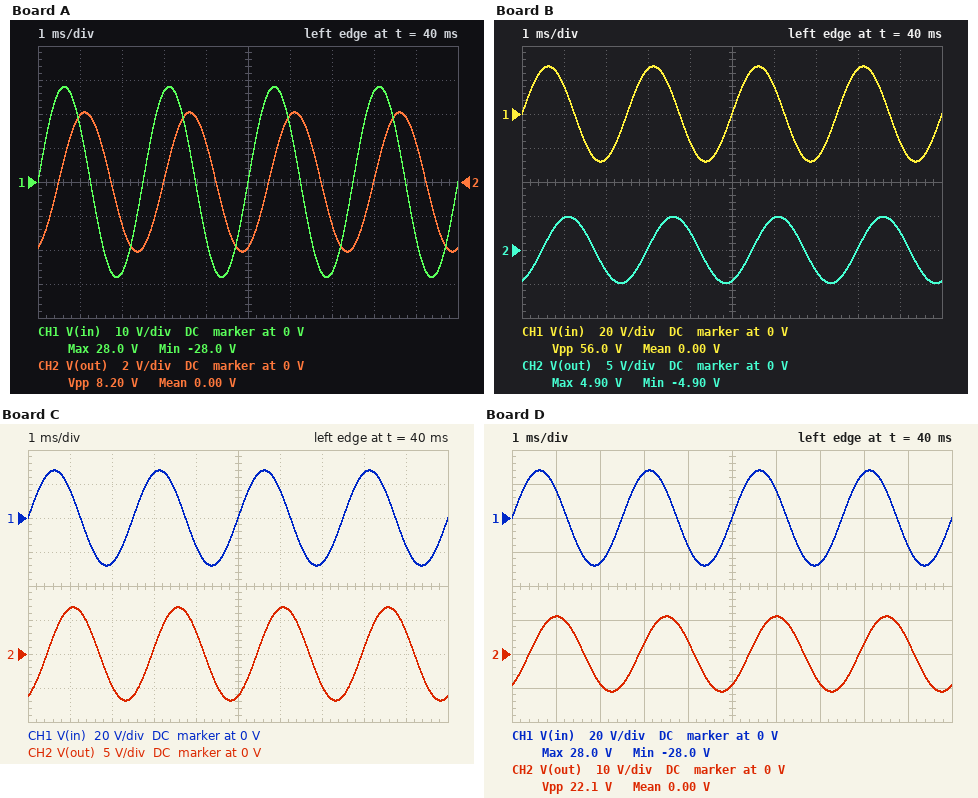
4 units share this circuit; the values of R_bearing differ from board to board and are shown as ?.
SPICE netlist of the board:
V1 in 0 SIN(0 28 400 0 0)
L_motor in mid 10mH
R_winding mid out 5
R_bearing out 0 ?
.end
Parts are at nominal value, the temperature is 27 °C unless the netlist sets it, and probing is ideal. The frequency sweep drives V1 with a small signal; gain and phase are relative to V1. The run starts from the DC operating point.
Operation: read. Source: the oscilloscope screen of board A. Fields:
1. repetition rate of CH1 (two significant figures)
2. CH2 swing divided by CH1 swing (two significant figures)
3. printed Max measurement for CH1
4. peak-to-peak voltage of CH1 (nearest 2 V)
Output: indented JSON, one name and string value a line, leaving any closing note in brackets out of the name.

{
  "repetition rate of CH1": "400 Hz",
  "CH2 swing divided by CH1 swing": "0.15",
  "printed Max measurement for CH1": "28.0 V",
  "peak-to-peak voltage of CH1": "56 V"
}
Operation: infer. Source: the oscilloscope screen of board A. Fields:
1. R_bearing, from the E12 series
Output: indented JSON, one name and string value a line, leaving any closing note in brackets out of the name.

{
  "R_bearing, from the E12 series": "3.9 Ω"
}
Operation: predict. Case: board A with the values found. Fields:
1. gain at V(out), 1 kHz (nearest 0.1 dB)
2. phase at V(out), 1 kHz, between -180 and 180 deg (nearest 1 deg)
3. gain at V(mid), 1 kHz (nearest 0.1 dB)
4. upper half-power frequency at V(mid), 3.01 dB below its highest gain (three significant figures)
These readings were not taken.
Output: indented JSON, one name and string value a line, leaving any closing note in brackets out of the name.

{
  "gain at V(out), 1 kHz": "-24.2 dB",
  "phase at V(out), 1 kHz, between -180 and 180 deg": "-82 deg",
  "gain at V(mid), 1 kHz": "-17.1 dB",
  "upper half-power frequency at V(mid), 3.01 dB below its highest gain": "142 Hz"
}
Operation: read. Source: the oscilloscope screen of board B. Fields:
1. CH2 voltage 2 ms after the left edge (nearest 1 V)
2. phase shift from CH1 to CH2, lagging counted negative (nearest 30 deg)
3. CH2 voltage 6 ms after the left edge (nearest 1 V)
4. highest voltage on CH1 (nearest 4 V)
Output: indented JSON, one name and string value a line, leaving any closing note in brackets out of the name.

{
  "CH2 voltage 2 ms after the left edge": "-3 V",
  "phase shift from CH1 to CH2, lagging counted negative": "-60 deg",
  "CH2 voltage 6 ms after the left edge": "5 V",
  "highest voltage on CH1": "28 V"
}
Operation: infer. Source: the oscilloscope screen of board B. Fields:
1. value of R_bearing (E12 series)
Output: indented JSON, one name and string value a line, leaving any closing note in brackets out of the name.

{
  "value of R_bearing": "4.7 Ω"
}
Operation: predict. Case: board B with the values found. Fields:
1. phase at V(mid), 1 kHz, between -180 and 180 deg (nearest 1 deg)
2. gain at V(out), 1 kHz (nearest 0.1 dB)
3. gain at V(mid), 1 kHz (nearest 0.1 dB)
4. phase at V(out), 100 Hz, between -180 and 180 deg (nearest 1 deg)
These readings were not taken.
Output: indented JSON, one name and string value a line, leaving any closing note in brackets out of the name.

{
  "phase at V(mid), 1 kHz, between -180 and 180 deg": "-81 deg",
  "gain at V(out), 1 kHz": "-22.6 dB",
  "gain at V(mid), 1 kHz": "-16.3 dB",
  "phase at V(out), 100 Hz, between -180 and 180 deg": "-33 deg"
}
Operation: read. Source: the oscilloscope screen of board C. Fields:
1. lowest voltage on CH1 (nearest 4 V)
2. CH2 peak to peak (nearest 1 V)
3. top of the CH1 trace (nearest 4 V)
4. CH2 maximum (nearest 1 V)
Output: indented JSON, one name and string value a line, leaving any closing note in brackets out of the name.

{
  "lowest voltage on CH1": "-28 V",
  "CH2 peak to peak": "14 V",
  "top of the CH1 trace": "28 V",
  "CH2 maximum": "7 V"
}
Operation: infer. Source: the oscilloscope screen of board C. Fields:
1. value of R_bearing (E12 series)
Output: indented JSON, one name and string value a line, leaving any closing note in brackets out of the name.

{
  "value of R_bearing": "6.8 Ω"
}
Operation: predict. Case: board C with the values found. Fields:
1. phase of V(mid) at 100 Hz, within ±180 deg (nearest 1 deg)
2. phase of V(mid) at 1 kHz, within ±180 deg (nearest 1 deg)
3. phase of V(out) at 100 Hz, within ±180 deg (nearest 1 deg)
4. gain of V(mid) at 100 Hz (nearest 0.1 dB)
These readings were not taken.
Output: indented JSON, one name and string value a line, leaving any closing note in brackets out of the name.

{
  "phase of V(mid) at 100 Hz, within ±180 deg": "-28 deg",
  "phase of V(mid) at 1 kHz, within ±180 deg": "-79 deg",
  "phase of V(out) at 100 Hz, within ±180 deg": "-28 deg",
  "gain of V(mid) at 100 Hz": "-1.1 dB"
}
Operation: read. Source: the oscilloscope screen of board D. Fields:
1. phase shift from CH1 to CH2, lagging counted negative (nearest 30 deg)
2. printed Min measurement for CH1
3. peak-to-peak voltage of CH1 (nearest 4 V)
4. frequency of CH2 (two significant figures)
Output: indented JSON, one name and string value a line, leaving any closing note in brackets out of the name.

{
  "phase shift from CH1 to CH2, lagging counted negative": "-60 deg",
  "printed Min measurement for CH1": "-28.0 V",
  "peak-to-peak voltage of CH1": "56 V",
  "frequency of CH2": "400 Hz"
}
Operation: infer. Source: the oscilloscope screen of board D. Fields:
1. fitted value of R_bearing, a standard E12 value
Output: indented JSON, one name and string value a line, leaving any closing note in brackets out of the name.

{
  "fitted value of R_bearing, a standard E12 value": "12 Ω"
}
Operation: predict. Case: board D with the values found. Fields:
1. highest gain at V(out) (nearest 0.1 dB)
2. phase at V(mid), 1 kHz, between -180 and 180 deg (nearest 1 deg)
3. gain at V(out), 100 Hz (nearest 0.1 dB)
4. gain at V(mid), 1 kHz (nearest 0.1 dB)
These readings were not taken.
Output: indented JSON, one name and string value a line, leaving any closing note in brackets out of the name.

{
  "highest gain at V(out)": "-3.0 dB",
  "phase at V(mid), 1 kHz, between -180 and 180 deg": "-75 deg",
  "gain at V(out), 100 Hz": "-3.6 dB",
  "gain at V(mid), 1 kHz": "-11.7 dB"
}
